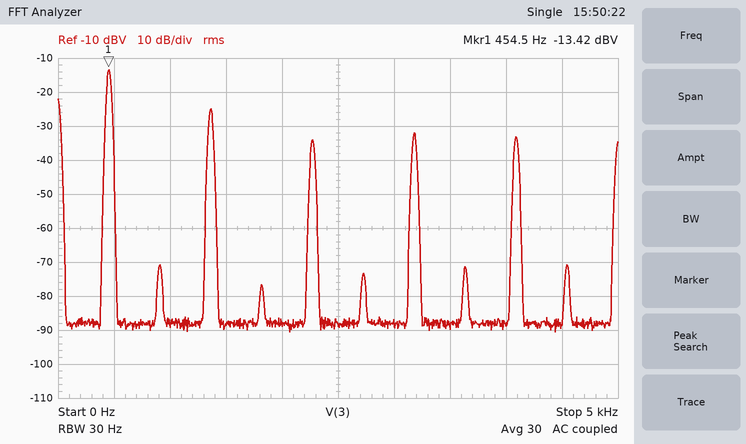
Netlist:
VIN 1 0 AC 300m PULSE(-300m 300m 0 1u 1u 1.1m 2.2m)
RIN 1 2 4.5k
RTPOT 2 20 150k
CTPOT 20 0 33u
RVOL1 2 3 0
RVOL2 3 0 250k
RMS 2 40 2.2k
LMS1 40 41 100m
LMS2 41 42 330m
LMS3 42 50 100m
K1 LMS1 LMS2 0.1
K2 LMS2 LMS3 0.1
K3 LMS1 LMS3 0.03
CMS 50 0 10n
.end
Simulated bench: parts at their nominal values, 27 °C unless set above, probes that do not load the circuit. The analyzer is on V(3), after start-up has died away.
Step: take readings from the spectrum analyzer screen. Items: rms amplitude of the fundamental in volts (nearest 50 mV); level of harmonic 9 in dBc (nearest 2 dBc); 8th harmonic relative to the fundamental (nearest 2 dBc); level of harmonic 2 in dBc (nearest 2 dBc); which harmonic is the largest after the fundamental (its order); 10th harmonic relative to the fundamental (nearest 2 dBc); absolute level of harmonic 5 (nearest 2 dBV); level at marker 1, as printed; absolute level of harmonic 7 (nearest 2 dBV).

200 mV
-20 dBc
-58 dBc
-58 dBc
3
-58 dBc
-34 dBV
-13.42 dBV
-32 dBV
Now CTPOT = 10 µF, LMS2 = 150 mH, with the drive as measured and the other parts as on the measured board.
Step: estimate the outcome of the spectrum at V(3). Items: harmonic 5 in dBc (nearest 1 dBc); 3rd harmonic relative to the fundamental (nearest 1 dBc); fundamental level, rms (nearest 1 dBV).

-21 dBc
-11 dBc
-13 dBV
